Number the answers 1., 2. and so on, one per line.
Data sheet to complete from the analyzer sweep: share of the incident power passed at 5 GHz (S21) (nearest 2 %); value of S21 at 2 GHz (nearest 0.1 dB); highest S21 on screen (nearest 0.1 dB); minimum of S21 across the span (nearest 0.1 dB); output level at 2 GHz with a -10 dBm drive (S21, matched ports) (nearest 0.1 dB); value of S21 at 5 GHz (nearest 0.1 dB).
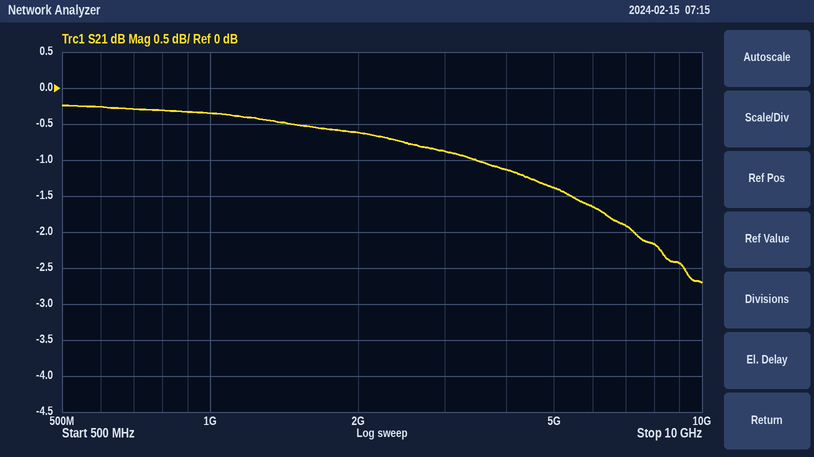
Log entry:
1. 72 %
2. -0.6 dB
3. -0.2 dB
4. -2.7 dB
5. -10.6 dBm
6. -1.4 dB
